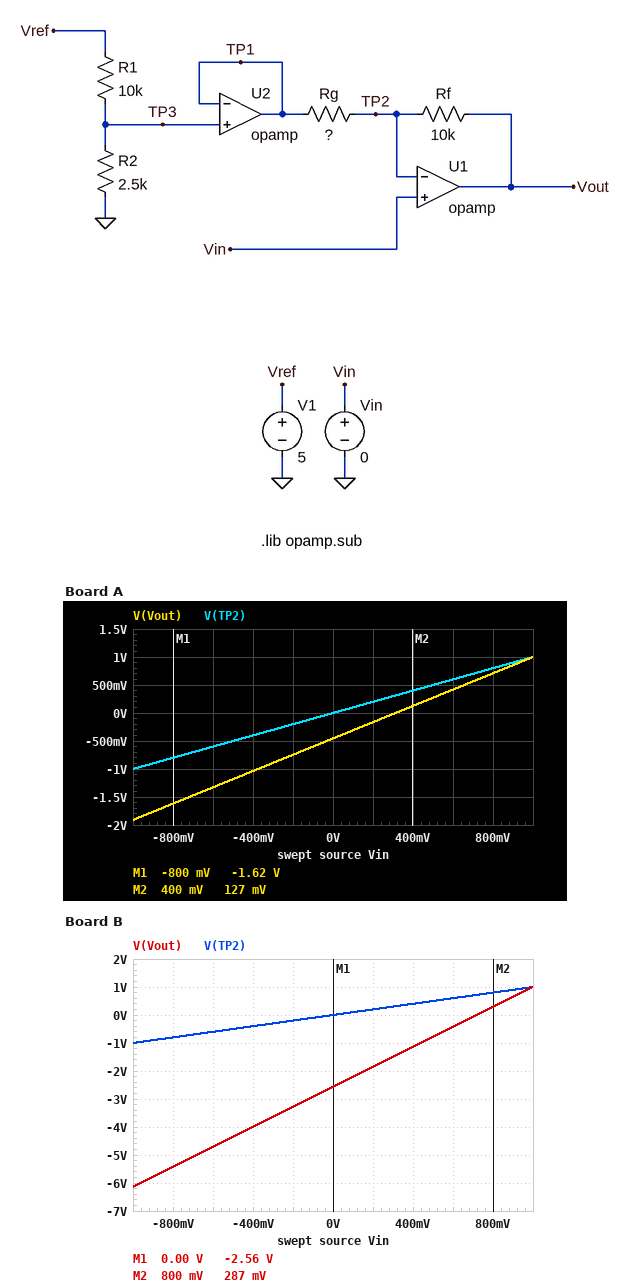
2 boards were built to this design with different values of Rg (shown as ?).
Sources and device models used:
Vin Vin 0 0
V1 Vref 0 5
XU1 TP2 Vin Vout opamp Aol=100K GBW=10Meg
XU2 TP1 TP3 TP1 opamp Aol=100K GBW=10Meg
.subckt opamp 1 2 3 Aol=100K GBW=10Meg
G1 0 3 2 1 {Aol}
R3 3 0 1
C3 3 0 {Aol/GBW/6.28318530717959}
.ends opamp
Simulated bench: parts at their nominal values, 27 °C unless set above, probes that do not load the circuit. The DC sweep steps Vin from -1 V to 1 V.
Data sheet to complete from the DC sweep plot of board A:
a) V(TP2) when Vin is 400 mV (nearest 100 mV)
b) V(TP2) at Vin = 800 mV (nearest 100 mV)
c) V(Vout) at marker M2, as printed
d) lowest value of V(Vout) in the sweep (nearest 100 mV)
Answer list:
400 mV
800 mV
127 mV
-1.9 V
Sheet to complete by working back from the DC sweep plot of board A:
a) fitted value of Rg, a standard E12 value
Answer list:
22 kΩ
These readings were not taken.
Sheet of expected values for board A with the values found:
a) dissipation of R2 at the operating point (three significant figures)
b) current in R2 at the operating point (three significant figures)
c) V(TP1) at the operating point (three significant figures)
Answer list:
400 µW
400 µA
1.00 V
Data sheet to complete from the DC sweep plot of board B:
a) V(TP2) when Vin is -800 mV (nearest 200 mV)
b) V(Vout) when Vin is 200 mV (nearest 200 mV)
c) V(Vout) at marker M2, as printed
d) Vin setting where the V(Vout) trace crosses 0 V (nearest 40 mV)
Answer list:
-800 mV
-1.8 V
287 mV
720 mV
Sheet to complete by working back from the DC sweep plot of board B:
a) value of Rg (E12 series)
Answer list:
3.9 kΩ
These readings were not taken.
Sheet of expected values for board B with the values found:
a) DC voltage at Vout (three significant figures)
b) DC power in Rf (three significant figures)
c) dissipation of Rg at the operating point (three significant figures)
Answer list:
-2.56 V
657 µW
256 µW
